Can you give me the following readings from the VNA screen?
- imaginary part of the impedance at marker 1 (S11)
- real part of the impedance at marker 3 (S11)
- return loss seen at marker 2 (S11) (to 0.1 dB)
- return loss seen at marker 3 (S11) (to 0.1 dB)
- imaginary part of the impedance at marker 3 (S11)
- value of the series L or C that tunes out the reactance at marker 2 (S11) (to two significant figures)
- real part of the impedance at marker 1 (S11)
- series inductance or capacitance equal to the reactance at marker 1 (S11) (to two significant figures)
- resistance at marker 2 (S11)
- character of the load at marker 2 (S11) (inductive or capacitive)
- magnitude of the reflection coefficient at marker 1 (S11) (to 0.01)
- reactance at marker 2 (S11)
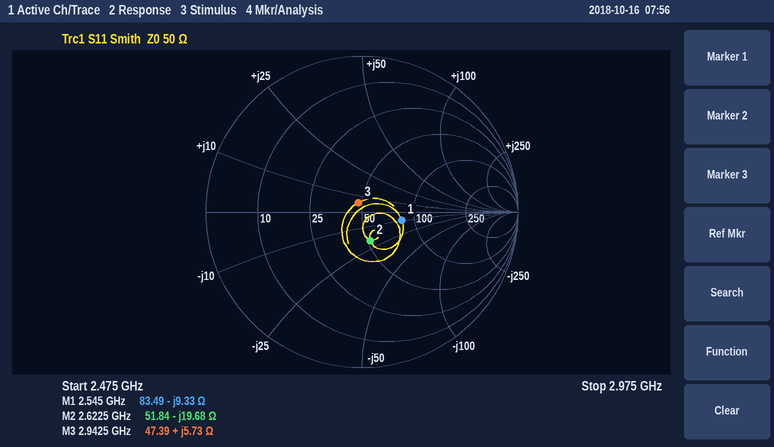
-9.33 Ω
47.39 Ω
14.4 dB
23.8 dB
+5.73 Ω
1.2 nH
83.49 Ω
6.7 pF
51.84 Ω
capacitive
0.26
-19.68 Ω
